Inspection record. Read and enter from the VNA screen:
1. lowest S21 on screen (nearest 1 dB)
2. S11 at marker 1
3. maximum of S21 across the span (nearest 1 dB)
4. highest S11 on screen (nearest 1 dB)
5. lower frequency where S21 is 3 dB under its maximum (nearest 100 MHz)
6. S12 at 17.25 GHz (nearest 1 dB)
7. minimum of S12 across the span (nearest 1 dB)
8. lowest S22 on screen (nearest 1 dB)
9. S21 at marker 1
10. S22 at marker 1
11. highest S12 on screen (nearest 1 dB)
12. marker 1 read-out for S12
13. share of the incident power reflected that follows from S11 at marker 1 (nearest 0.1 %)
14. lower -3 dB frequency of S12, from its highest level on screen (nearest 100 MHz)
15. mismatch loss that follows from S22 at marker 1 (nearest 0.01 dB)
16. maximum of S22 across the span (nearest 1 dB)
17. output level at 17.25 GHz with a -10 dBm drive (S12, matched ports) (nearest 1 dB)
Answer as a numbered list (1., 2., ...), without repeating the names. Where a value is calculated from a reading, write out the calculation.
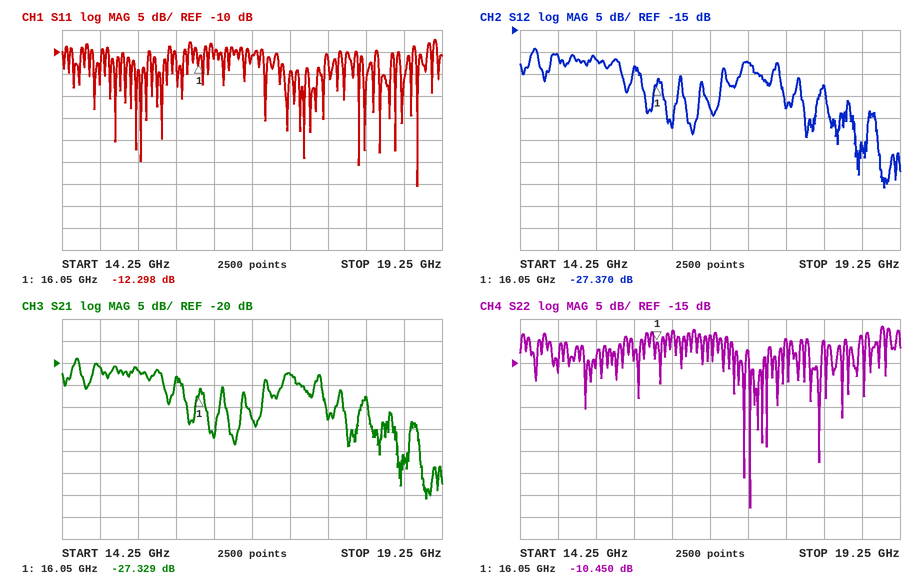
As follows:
1. -51 dB
2. -12.298 dB
3. -19 dB
4. -7 dB
5. 14.4 GHz
6. -22 dB
7. -51 dB
8. -48 dB
9. -27.329 dB
10. -10.450 dB
11. -19 dB
12. -27.370 dB
13. 10^(-12.298/10) ≈ 5.9 %
14. 14.4 GHz
15. −10 log10(1 − 10^(-10.45/10)) ≈ 0.41 dB
16. -7 dB
17. -10 dBm + (-22 dB) = -32 dBm
